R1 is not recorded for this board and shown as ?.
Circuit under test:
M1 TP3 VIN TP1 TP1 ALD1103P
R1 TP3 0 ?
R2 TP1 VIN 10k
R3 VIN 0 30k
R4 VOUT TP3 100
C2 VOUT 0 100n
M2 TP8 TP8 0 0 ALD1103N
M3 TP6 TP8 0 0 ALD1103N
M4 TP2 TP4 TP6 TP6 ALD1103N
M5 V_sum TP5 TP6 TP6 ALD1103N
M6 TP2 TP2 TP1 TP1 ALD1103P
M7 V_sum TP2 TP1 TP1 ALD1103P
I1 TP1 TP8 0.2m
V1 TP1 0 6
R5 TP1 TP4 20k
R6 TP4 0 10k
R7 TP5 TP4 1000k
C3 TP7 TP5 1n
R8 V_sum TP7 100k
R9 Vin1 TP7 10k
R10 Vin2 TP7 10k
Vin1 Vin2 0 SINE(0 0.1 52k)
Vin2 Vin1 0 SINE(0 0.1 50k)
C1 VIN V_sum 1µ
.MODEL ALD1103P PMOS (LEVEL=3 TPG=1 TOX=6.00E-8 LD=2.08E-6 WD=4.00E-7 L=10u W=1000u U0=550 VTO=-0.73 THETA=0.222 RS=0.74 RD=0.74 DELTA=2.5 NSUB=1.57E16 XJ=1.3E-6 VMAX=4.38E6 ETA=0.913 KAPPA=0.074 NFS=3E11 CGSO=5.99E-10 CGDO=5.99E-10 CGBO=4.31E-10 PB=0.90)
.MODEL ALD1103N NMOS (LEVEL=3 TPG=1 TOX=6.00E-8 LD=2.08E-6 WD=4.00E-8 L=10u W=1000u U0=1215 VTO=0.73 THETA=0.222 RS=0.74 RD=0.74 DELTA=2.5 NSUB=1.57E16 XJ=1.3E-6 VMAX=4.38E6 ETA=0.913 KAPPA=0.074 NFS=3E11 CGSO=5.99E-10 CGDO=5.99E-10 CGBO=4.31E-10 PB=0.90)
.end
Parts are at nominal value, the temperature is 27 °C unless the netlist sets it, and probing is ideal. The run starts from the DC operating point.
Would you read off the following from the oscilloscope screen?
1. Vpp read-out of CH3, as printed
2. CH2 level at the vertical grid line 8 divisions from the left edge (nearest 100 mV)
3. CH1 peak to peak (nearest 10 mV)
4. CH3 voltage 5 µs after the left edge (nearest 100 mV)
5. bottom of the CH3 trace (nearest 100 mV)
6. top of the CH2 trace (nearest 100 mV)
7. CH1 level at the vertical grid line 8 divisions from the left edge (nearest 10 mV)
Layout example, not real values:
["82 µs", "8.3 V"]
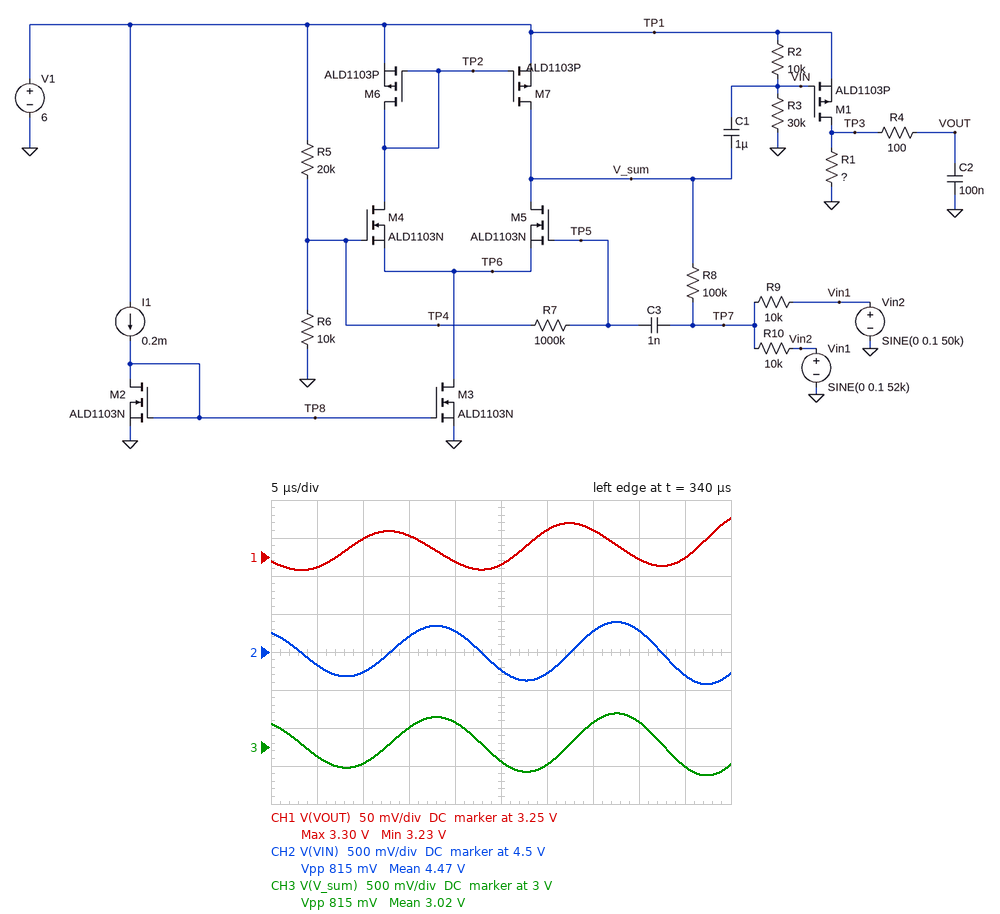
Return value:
["815 mV", "4.8 V", "70 mV", "2.9 V", "2.6 V", "4.9 V", "3.25 V"]
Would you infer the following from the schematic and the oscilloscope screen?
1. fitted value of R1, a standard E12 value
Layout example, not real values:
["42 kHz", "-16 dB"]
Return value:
["2.7 kΩ"]
